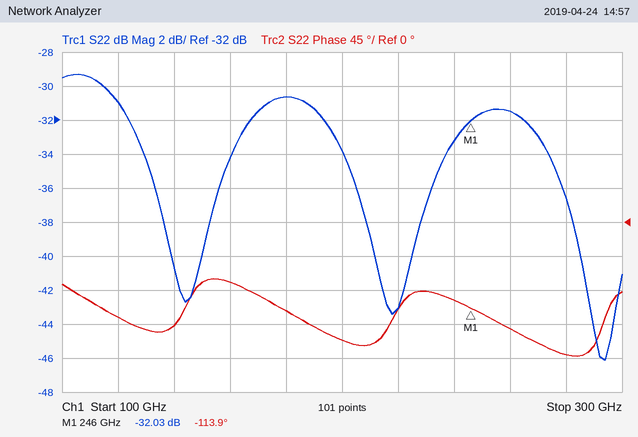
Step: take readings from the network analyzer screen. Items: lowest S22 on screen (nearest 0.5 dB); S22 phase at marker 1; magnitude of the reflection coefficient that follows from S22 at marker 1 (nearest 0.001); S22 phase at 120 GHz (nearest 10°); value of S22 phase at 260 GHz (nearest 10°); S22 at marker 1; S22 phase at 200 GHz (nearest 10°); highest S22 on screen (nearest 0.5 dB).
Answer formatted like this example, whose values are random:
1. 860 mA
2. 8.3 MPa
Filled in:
1. -46.0 dB
2. -113.9°
3. 0.025
4. -130°
5. -140°
6. -32.03 dB
7. -160°
8. -29.5 dB
